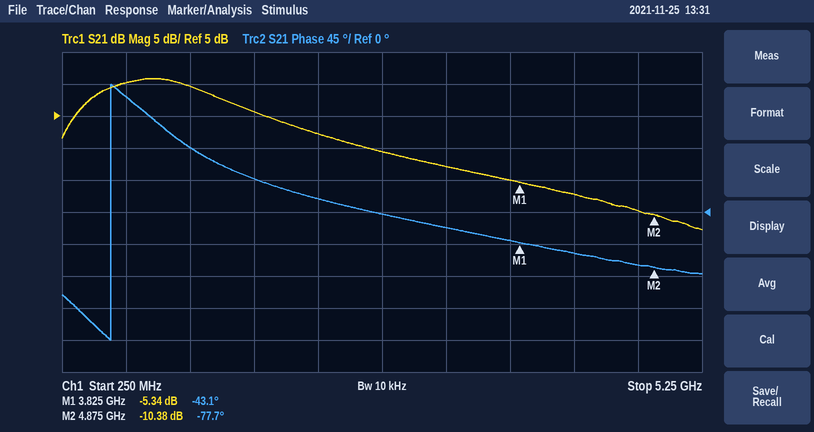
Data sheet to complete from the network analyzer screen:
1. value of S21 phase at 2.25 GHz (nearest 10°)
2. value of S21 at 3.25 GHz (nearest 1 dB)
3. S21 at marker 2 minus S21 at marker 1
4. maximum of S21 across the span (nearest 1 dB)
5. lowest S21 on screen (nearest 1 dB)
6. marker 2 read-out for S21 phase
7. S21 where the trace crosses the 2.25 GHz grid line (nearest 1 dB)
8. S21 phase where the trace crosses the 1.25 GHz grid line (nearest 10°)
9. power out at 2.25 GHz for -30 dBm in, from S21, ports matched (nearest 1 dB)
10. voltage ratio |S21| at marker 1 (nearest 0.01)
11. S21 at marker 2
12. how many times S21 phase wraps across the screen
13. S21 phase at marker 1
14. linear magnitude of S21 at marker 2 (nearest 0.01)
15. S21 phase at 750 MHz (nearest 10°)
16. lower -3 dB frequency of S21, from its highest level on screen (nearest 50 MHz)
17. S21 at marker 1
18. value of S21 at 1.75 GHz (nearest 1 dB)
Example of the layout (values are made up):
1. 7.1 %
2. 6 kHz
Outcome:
1. 20°
2. -3 dB
3. -5.04 dB
4. 11 dB
5. -13 dB
6. -77.7°
7. 2 dB
8. 90°
9. -28 dBm
10. 0.54
11. -10.38 dB
12. 1
13. -43.1°
14. 0.30
15. 160°
16. 500 MHz
17. -5.34 dB
18. 6 dB
